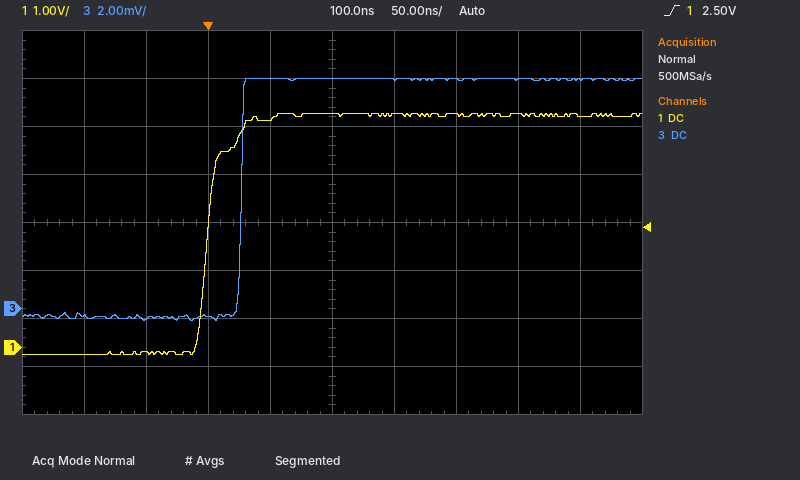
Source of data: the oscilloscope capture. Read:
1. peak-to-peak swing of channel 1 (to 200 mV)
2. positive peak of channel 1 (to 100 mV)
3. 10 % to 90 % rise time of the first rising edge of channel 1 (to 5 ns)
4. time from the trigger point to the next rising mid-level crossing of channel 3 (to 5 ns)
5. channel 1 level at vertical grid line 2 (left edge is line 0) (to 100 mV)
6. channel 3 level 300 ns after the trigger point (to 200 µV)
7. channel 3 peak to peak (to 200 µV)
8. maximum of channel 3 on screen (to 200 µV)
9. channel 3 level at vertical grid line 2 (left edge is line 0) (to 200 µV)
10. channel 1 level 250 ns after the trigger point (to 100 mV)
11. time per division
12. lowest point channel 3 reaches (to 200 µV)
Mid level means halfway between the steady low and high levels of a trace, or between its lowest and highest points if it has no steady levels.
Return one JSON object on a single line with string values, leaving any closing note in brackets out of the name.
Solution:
{"peak-to-peak swing of channel 1": "5.0 V", "positive peak of channel 1": "4.9 V", "10 % to 90 % rise time of the first rising edge of channel 1": "30 ns", "time from the trigger point to the next rising mid-level crossing of channel 3": "25 ns", "channel 1 level at vertical grid line 2 (left edge is line 0)": "-100 mV", "channel 3 level 300 ns after the trigger point": "9.6 mV", "channel 3 peak to peak": "10.0 mV", "maximum of channel 3 on screen": "9.6 mV", "channel 3 level at vertical grid line 2 (left edge is line 0)": "-400 µV", "channel 1 level 250 ns after the trigger point": "4.9 V", "time per division": "50 ns", "lowest point channel 3 reaches": "-400 µV"}
